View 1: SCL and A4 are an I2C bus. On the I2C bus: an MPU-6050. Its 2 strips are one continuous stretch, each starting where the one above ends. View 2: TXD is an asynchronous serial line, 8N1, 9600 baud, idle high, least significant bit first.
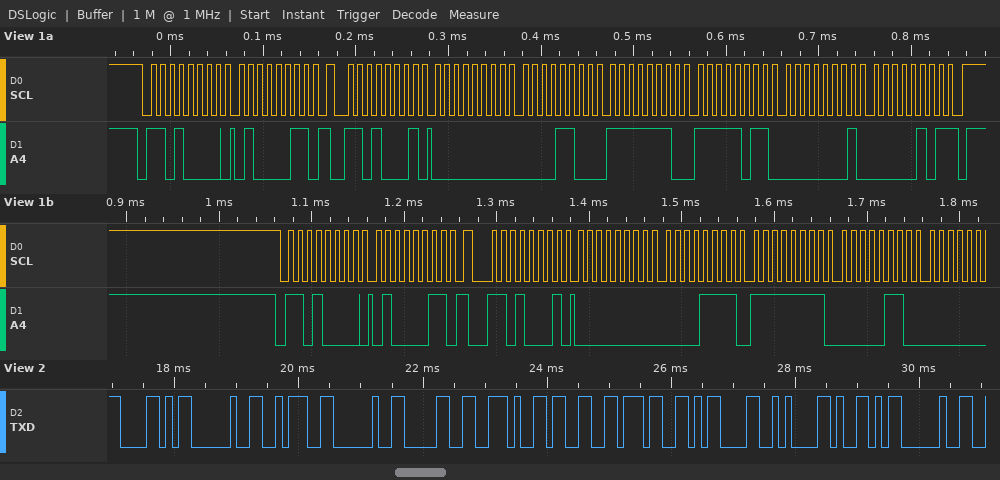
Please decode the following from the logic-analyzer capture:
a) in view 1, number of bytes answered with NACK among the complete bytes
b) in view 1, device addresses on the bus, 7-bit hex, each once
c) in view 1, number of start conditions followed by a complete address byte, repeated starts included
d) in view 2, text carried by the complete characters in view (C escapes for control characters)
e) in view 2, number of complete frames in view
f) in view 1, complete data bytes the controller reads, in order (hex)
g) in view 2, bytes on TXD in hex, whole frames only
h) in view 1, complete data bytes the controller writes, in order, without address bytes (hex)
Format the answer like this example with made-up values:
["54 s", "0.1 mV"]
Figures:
["1", "0x68", "4", "\"X : 0.37\\r\\nY \"", "12", "00 0C FE FB 01 05 00 0F FF 06", "58 20 3A 20 30 2E 33 37 0D 0A 59 20", "43 43"]
